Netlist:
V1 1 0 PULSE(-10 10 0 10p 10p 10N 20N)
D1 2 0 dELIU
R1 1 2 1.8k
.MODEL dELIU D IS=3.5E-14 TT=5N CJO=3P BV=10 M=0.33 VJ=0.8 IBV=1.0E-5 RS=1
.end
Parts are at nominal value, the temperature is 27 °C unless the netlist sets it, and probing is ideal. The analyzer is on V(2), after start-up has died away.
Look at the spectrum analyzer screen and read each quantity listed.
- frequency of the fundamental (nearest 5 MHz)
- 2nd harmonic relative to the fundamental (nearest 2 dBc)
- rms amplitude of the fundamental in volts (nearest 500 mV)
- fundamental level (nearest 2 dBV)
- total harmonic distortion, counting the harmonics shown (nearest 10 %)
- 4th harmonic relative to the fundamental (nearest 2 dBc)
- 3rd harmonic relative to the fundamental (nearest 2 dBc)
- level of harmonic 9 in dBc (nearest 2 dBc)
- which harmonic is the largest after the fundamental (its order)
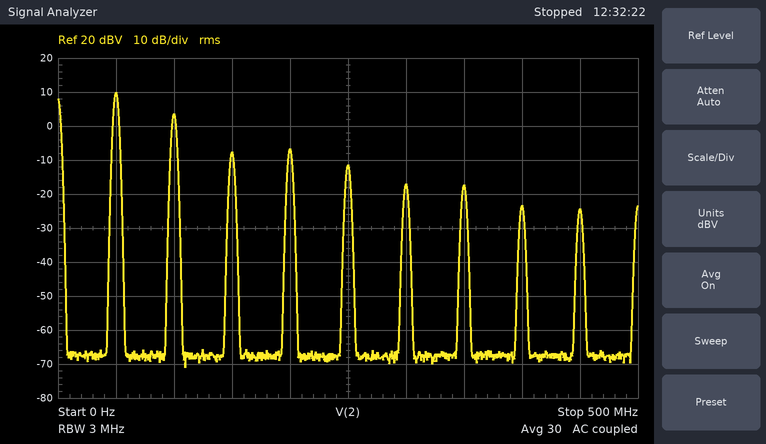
50 MHz
-6 dBc
3.0 V
10 dBV
50 %
-16 dBc
-18 dBc
-34 dBc
2
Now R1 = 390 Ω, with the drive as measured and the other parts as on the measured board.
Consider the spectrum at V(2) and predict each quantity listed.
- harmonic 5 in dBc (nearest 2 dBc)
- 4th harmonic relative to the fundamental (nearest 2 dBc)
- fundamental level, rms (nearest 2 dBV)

-16 dBc
-12 dBc
12 dBV
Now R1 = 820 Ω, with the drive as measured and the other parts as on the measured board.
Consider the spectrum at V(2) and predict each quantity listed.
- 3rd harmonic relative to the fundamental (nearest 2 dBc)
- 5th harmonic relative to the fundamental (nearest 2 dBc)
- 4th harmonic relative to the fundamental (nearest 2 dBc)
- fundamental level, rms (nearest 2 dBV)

-22 dBc
-18 dBc
-14 dBc
12 dBV
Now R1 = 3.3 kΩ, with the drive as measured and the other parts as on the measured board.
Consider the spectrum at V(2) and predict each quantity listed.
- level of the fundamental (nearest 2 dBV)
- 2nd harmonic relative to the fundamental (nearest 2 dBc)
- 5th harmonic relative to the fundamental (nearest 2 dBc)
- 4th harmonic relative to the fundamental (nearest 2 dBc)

8 dBV
-8 dBc
-28 dBc
-20 dBc
